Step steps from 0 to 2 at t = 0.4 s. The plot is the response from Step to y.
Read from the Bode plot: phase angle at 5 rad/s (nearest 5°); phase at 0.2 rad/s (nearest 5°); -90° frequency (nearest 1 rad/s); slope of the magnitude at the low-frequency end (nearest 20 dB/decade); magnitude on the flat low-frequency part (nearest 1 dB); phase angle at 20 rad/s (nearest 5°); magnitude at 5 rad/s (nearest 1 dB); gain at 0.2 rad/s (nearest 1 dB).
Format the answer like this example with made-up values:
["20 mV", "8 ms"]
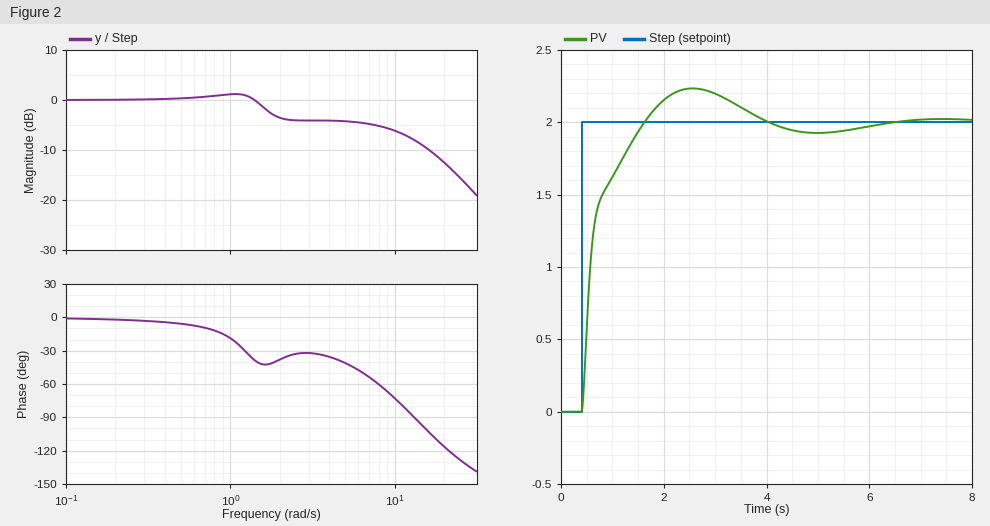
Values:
["-40°", "0°", "13 rad/s", "0 dB/decade", "0 dB", "-115°", "-4 dB", "0 dB"]
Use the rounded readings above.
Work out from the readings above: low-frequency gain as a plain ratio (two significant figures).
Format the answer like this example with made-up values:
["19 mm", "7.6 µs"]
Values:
["1.0"]
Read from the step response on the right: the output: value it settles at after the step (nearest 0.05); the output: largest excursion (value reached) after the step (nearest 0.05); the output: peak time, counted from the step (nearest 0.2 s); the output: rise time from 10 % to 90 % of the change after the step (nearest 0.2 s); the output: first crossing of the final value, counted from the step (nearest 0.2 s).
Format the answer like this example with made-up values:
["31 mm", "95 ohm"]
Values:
["2.00", "2.25", "2.2 s", "0.8 s", "1.2 s"]
